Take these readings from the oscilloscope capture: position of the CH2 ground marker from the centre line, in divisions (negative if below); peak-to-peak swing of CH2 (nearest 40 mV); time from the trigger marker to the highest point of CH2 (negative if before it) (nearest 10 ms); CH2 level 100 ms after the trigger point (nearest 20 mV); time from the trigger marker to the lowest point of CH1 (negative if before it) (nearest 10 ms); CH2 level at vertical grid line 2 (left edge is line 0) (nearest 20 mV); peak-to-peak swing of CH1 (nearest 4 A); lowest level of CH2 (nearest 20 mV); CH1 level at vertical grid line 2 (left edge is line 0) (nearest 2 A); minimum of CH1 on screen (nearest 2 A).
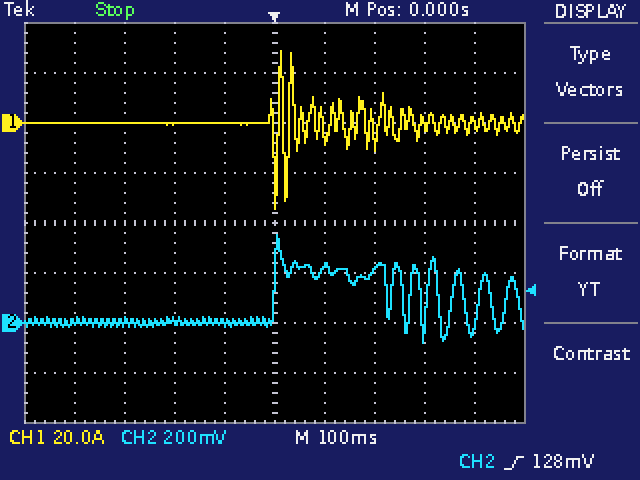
-2.0 div
440 mV
+10 ms
220 mV
0 ms
0 mV
64 A
-80 mV
0 A
-34 A
